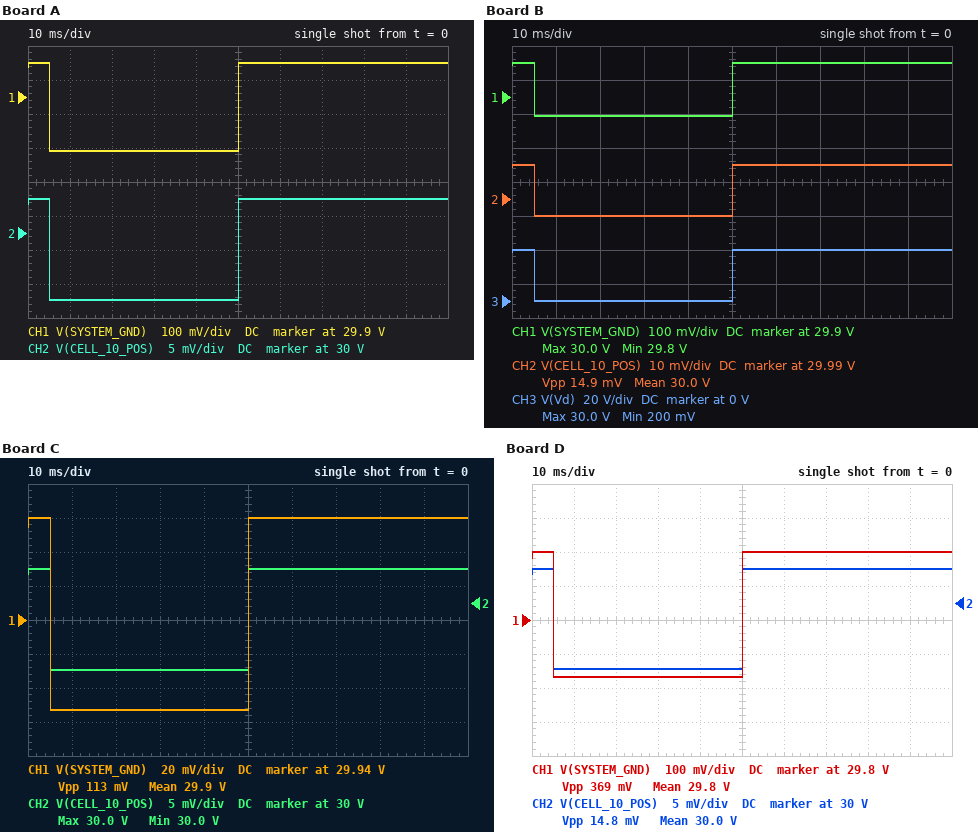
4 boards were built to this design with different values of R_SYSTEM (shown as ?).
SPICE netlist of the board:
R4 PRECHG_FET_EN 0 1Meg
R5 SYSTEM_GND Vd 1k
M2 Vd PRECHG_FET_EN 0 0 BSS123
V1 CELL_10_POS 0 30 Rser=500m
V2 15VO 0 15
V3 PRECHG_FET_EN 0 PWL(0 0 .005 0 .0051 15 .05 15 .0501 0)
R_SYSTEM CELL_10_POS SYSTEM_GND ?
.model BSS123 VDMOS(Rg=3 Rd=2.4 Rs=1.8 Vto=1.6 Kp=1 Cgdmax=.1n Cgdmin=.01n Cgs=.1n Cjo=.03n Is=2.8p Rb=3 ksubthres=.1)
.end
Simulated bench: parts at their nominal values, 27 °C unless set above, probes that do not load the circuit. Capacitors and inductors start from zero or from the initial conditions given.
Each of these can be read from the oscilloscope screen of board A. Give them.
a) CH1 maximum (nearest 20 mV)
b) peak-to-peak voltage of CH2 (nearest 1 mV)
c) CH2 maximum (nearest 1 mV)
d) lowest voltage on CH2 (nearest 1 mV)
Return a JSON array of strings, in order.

["30.00 V", "15 mV", "30.000 V", "29.985 V"]
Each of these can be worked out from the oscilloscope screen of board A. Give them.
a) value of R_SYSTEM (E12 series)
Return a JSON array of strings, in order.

["8.2 Ω"]
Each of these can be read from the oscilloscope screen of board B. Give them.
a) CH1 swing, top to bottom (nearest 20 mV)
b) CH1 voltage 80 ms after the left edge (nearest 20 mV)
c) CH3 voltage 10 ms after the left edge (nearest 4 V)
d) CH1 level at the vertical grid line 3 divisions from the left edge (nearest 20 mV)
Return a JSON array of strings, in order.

["160 mV", "30.00 V", "0 V", "29.84 V"]
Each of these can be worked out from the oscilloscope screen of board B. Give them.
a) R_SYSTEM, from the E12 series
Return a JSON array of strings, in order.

["4.7 Ω"]
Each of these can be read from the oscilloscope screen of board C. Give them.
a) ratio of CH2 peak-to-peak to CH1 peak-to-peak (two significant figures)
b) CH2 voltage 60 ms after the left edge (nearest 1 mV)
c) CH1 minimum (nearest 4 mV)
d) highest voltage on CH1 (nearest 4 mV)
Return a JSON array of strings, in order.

["0.13", "30.000 V", "29.888 V", "30.000 V"]
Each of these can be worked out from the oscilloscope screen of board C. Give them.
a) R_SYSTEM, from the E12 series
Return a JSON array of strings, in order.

["3.3 Ω"]
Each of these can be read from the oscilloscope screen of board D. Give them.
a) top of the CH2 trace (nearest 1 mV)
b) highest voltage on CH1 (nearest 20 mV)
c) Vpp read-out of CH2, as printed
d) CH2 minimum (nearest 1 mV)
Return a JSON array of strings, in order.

["30.000 V", "30.00 V", "14.8 mV", "29.985 V"]
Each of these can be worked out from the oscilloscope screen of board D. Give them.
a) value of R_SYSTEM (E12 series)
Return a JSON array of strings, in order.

["12 Ω"]
